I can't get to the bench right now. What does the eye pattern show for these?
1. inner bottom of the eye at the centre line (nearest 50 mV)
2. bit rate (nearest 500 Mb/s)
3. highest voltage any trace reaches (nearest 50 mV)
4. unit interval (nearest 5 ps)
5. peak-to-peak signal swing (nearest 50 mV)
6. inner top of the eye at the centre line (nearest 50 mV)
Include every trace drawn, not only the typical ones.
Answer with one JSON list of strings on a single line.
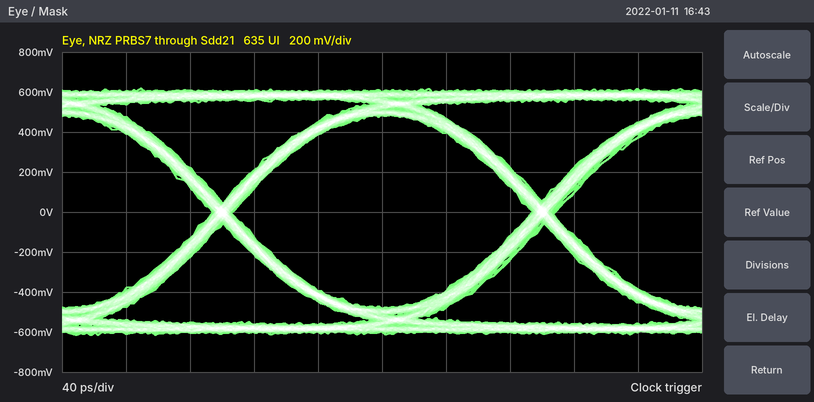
["-500 mV", "5.0 Gb/s", "600 mV", "200 ps", "1.25 V", "500 mV"]
